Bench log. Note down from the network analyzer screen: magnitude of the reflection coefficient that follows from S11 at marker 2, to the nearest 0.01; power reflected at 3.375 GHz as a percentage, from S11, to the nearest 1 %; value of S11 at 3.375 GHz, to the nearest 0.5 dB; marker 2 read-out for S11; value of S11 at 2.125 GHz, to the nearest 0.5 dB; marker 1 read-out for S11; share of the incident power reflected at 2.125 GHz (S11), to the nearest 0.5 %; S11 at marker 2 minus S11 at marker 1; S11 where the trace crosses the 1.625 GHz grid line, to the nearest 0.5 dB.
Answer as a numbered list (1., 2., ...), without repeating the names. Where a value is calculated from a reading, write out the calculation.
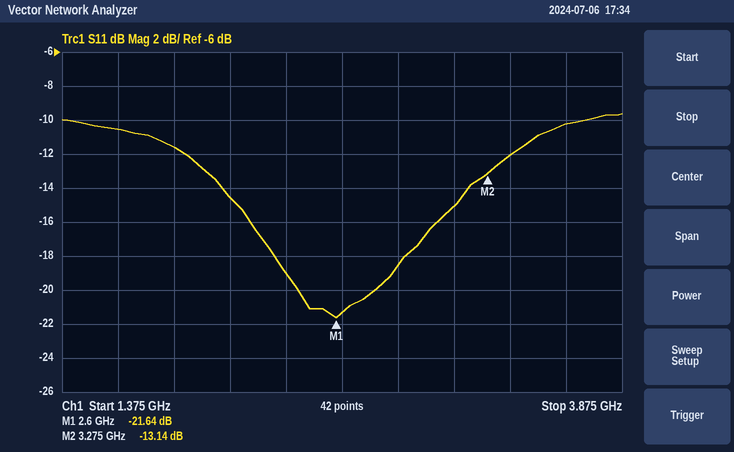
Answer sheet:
1. 10^(-13.14/20) ≈ 0.22
2. 10^(-12/10) ≈ 6 %
3. -12.0 dB
4. -13.14 dB
5. -14.5 dB
6. -21.64 dB
7. 10^(-14.5/10) ≈ 3.5 %
8. -13.14 − (-21.64) = 8.50 dB
9. -10.5 dB
